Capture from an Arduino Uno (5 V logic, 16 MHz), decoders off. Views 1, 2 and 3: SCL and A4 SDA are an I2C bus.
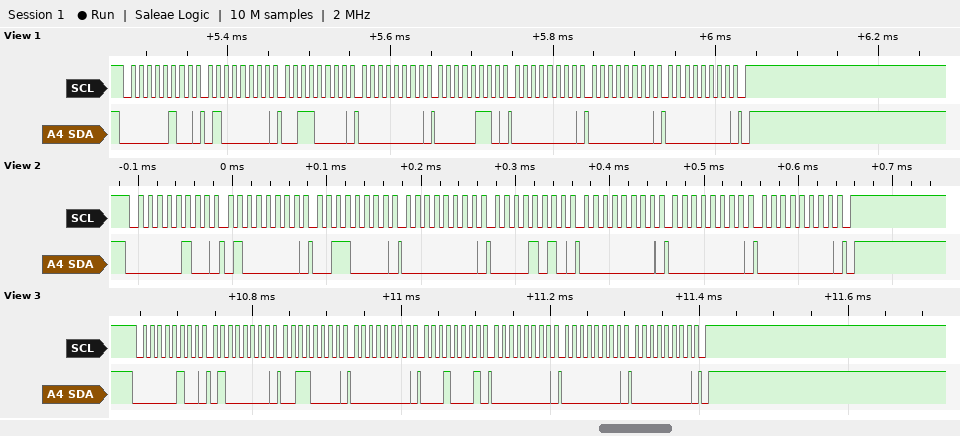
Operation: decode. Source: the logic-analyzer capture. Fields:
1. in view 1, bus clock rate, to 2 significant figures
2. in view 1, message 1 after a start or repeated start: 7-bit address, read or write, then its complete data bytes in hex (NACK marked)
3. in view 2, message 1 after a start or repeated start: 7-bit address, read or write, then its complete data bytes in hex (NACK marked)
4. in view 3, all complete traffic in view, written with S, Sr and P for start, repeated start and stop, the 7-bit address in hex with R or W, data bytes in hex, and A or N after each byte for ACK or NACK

100 kHz
0x02 write: 40 30 00 06 00 00 00
0x02 write: 40 30 00 0A 00 00 00
S 02W A 40 A 30 A 00 A 11 A 00 A 00 A 00 A P
